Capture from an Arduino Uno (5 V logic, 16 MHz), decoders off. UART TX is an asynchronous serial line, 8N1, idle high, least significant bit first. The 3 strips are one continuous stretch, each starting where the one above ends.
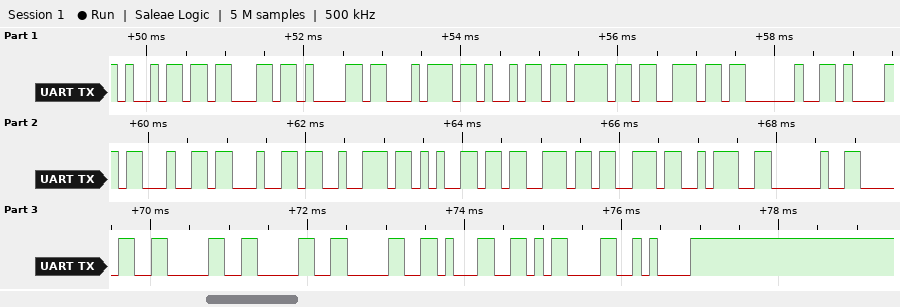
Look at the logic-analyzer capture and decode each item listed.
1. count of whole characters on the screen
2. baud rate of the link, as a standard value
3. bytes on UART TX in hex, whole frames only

24
9600 baud
0x69 0x63 0x61 0x74 0x69 0x6F 0x6E 0x20 0x61 0x64 0x64 0x72 0x65 0x73 0x73 0x3A 0x20 0x30 0x30 0x30 0x30 0x31 0x0D 0x0A
